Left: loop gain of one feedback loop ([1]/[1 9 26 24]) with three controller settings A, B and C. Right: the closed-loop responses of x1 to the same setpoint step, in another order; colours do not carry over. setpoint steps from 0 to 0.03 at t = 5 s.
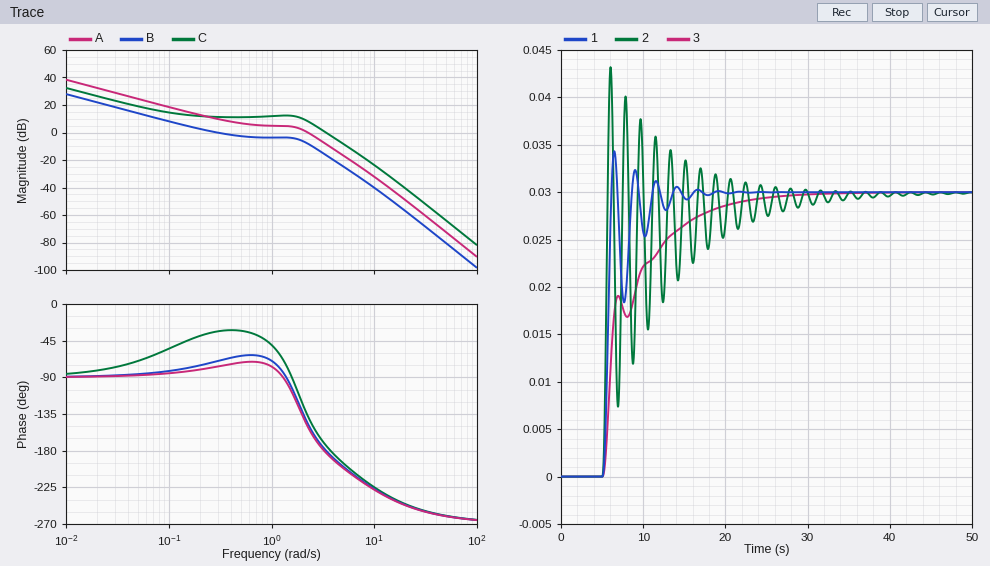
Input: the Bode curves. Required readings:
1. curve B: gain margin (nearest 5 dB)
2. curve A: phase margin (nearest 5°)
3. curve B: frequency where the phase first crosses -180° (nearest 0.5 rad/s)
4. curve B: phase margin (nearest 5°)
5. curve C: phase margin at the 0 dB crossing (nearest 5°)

15 dB
30°
3.5 rad/s
110°
5°
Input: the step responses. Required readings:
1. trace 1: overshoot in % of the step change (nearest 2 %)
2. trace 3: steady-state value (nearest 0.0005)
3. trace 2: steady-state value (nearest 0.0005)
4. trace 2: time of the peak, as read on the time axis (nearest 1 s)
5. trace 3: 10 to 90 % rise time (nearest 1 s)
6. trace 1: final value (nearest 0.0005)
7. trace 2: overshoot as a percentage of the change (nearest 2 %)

14 %
0.0300
0.0300
6 s
10 s
0.0300
44 %
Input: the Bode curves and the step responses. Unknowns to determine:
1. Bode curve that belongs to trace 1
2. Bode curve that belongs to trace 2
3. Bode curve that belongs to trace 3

A
C
B
